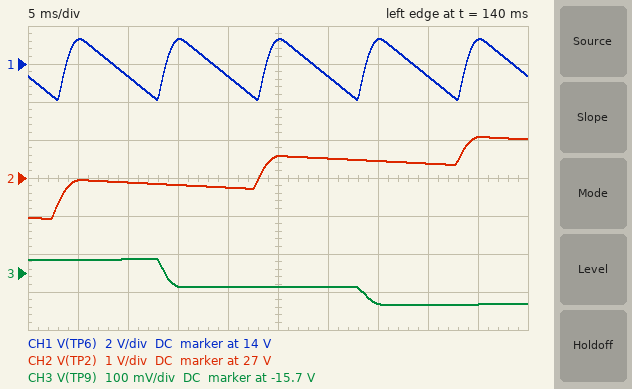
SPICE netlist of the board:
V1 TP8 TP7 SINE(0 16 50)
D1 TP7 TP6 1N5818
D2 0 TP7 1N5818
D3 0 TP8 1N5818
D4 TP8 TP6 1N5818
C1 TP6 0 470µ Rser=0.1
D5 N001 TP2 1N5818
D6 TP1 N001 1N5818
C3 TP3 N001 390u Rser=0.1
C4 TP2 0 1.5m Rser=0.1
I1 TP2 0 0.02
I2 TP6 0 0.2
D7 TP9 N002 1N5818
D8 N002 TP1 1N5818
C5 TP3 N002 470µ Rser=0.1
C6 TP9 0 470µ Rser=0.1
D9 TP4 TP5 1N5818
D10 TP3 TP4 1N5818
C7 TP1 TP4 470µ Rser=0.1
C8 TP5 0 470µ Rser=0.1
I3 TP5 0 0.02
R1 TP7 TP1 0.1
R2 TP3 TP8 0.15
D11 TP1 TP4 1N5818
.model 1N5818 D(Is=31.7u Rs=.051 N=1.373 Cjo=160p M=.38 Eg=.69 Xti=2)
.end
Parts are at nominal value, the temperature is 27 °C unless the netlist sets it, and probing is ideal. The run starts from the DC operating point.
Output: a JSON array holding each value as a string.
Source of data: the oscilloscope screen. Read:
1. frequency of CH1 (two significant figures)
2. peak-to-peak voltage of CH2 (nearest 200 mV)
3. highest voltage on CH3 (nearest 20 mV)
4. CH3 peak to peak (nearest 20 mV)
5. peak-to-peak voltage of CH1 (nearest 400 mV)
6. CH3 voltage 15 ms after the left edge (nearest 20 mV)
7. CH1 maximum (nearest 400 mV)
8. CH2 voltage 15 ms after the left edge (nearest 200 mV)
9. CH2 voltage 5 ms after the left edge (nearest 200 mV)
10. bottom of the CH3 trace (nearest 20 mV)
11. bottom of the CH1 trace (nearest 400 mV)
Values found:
["100 Hz", "2.2 V", "-15.66 V", "120 mV", "3.2 V", "-15.74 V", "15.2 V", "26.8 V", "27.0 V", "-15.78 V", "12.0 V"]
